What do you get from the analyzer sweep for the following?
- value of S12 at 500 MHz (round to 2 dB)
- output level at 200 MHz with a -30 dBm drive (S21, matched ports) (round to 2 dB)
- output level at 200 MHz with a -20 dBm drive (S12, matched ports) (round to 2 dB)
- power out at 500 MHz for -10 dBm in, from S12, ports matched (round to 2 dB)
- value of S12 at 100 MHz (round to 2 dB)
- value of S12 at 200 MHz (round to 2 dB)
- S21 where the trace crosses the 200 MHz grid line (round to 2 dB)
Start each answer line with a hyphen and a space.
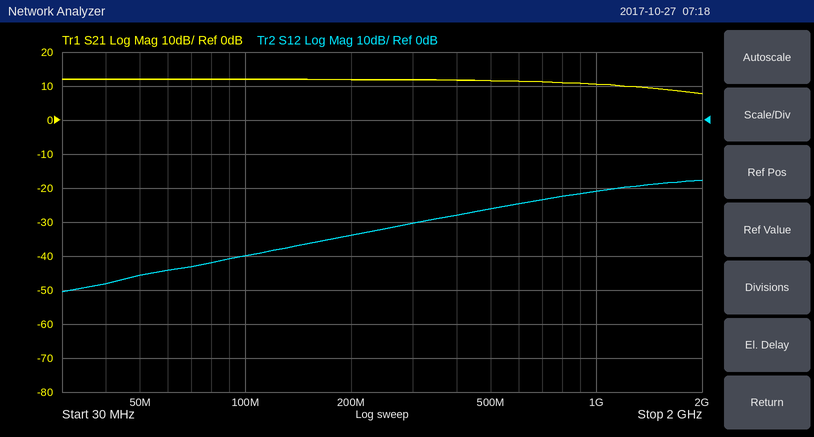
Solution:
- -26 dB
- -18 dBm
- -54 dBm
- -36 dBm
- -40 dB
- -34 dB
- 12 dB
